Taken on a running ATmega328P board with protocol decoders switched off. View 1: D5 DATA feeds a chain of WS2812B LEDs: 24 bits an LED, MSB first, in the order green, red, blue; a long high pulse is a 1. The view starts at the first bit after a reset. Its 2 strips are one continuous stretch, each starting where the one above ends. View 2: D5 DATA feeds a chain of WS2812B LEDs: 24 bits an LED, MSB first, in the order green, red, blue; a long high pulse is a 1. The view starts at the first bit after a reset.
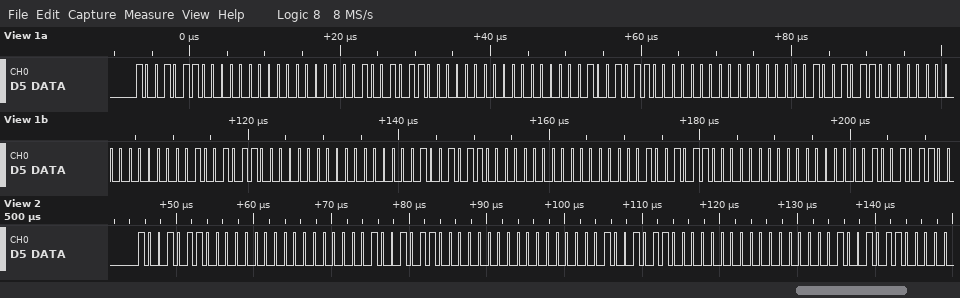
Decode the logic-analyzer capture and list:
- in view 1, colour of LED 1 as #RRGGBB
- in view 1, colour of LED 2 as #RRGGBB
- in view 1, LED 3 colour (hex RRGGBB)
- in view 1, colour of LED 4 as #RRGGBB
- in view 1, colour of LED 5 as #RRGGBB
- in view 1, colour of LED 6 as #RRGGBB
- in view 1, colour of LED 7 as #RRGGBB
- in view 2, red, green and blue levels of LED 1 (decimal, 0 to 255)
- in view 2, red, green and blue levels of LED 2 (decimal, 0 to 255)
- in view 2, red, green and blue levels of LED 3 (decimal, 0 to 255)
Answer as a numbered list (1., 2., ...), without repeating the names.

1. #009600
2. #009600
3. #009600
4. #009600
5. #009600
6. #009600
7. #009600
8. 0, 150, 0
9. 0, 150, 0
10. 0, 150, 0
